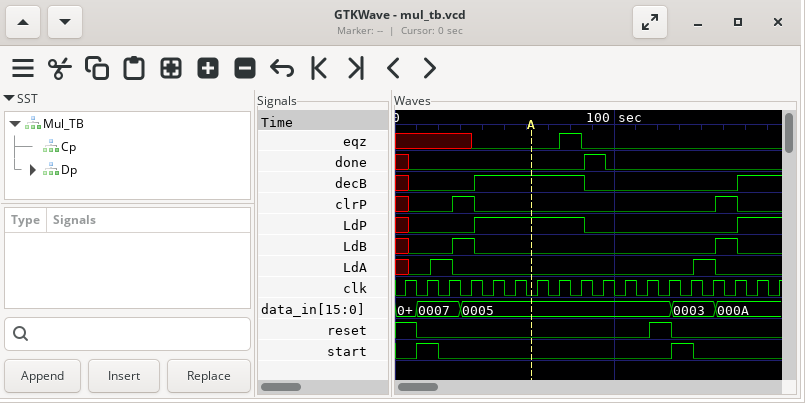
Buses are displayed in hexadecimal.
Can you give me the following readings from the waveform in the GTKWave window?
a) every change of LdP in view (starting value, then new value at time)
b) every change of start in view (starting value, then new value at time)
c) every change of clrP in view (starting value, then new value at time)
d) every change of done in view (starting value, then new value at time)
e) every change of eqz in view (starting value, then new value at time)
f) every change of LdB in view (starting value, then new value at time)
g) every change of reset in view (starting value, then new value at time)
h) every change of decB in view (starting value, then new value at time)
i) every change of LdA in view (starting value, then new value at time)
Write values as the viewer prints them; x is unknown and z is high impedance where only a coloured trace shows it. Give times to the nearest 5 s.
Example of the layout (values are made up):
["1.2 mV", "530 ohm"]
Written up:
["x, 0 at 5 s, 1 at 35 s, 0 at 85 s, 1 at 155 s", "0, 1 at 10 s, 0 at 20 s, 1 at 125 s, 0 at 135 s", "x, 0 at 5 s, 1 at 25 s, 0 at 35 s, 1 at 145 s, 0 at 155 s", "x, 0 at 5 s, 1 at 85 s, 0 at 95 s", "x, 0 at 35 s, 1 at 75 s, 0 at 85 s", "x, 0 at 5 s, 1 at 25 s, 0 at 35 s, 1 at 145 s, 0 at 155 s", "1, 0 at 10 s, 1 at 115 s, 0 at 125 s", "x, 0 at 5 s, 1 at 35 s, 0 at 85 s, 1 at 155 s", "x, 0 at 5 s, 1 at 15 s, 0 at 25 s, 1 at 135 s, 0 at 145 s"]
